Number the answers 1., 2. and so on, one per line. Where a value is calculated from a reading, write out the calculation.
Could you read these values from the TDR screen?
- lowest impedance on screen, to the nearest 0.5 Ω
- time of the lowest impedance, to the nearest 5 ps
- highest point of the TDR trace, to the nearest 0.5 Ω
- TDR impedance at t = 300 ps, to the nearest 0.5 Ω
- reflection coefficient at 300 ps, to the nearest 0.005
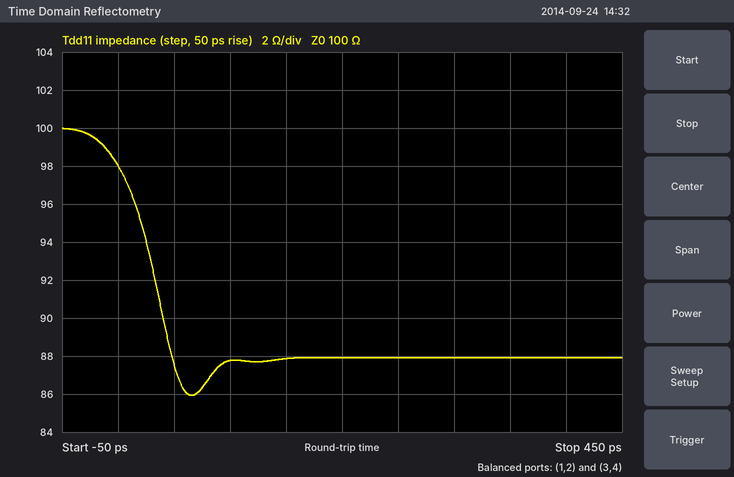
1. 86.0 Ω
2. 65 ps
3. 100.0 Ω
4. 88.0 Ω
5. (88 − 100)/(88 + 100) ≈ -0.0638, so -0.065 to the nearest 0.005
